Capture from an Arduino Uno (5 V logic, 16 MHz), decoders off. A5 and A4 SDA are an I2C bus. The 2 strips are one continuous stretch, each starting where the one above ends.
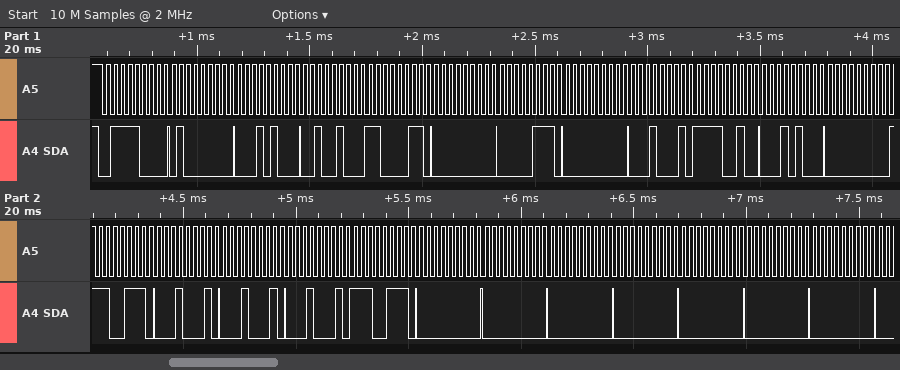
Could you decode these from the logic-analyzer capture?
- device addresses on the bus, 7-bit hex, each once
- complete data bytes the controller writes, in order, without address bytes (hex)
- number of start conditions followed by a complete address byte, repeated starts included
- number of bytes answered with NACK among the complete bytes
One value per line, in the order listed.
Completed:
0x3C
40 14 24 C3 00 07 00 11 F2 14 00 E7 11 11 11 E7 00 00 00 00 00 00 00
1
0
